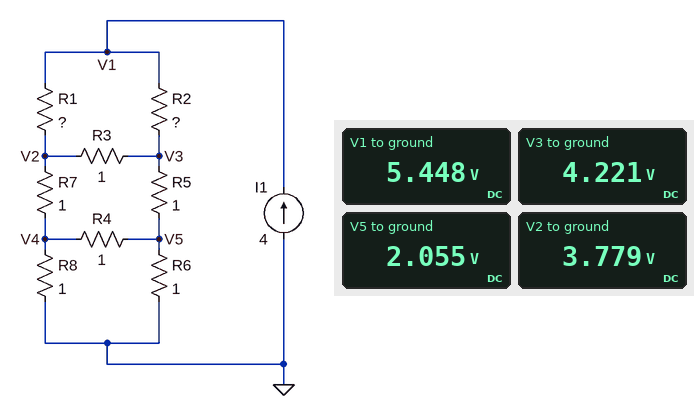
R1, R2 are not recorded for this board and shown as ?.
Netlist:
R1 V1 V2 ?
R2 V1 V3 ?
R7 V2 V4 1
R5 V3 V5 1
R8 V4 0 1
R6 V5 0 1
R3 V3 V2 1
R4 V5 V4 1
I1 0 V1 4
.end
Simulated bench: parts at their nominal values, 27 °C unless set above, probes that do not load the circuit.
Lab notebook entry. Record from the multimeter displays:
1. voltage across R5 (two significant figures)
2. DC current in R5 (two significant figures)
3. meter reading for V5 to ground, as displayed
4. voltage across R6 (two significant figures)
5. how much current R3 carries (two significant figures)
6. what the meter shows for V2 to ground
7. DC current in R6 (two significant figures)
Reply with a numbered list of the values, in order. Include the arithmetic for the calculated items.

1. 4.221 V - 2.055 V = 2.2 V
2. (4.221 V - 2.055 V) / 1 Ω = 2.2 A
3. 2.055 V
4. 2.055 V = 2.1 V
5. (4.221 V - 3.779 V) / 1 Ω = 440 mA
6. 3.779 V
7. (2.055 V) / 1 Ω = 2.1 A
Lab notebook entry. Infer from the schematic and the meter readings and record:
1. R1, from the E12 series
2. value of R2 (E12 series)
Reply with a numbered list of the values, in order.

1. 1.2 Ω
2. 0.47 Ω
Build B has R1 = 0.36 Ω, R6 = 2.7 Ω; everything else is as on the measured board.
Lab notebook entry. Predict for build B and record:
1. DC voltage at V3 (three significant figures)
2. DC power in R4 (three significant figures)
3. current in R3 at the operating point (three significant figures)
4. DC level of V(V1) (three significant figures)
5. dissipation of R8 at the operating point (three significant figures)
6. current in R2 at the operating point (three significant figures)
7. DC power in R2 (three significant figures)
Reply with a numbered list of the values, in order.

1. 5.04 V
2. 269 mW
3. 2.15 mA
4. 5.85 V
5. 7.72 W
6. 1.74 A
7. 1.42 W
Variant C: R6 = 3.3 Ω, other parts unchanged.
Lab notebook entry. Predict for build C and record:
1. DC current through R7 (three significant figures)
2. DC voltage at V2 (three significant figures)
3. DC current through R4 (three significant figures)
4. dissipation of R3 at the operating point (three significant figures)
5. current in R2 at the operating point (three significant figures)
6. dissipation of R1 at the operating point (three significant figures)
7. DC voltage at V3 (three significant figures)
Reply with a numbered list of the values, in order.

1. 2.09 A
2. 4.98 V
3. 792 mA
4. 366 mW
5. 2.51 A
6. 2.66 W
7. 5.58 V
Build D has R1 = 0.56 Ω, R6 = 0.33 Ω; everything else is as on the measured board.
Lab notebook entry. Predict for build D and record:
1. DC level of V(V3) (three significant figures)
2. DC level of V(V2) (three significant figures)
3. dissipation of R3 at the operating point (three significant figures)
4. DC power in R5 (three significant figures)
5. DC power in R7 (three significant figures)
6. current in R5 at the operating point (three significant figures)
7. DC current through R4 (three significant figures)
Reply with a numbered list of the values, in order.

1. 3.10 V
2. 3.12 V
3. 430 µW
4. 4.91 W
5. 3.18 W
6. 2.22 A
7. 452 mA
